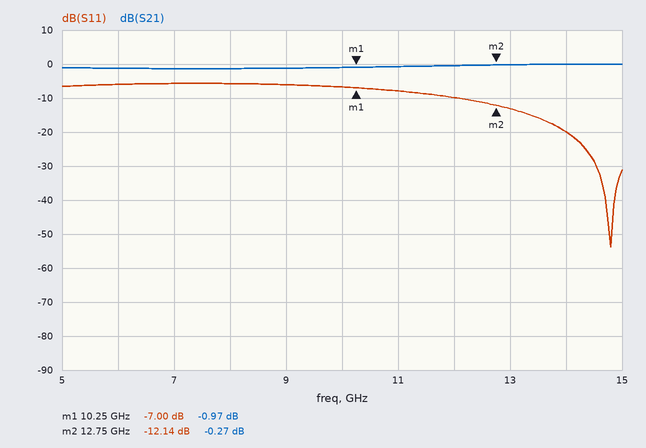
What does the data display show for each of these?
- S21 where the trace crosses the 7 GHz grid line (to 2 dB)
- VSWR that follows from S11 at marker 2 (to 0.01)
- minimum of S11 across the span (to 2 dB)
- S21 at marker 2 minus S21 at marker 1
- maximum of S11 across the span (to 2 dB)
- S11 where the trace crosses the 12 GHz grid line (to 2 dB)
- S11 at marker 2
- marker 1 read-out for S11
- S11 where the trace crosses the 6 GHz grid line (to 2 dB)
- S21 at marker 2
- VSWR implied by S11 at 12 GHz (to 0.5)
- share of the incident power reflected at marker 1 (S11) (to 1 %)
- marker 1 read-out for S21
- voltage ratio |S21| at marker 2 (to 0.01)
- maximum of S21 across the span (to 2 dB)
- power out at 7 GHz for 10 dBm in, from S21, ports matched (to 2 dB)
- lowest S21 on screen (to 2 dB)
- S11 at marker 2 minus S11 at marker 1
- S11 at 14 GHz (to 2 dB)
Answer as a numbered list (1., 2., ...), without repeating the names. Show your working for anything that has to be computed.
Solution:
1. -2 dB
2. (1 + 0.2472)/(1 − 0.2472) ≈ 1.66
3. -54 dB
4. -0.27 − (-0.97) = 0.70 dB
5. -6 dB
6. -10 dB
7. -12.14 dB
8. -7.00 dB
9. -6 dB
10. -0.27 dB
11. |Γ| = 10^(-10/20) = 0.3162; VSWR = (1 + 0.3162)/(1 − 0.3162) ≈ 1.92, so 2.0 to the nearest 0.5
12. 10^(-7/10) ≈ 20 %
13. -0.97 dB
14. 10^(-0.27/20) ≈ 0.97
15. 0 dB
16. 10 dBm + (-2 dB) = 8 dBm
17. -2 dB
18. -12.14 − (-7) = -5.14 dB
19. -20 dB
